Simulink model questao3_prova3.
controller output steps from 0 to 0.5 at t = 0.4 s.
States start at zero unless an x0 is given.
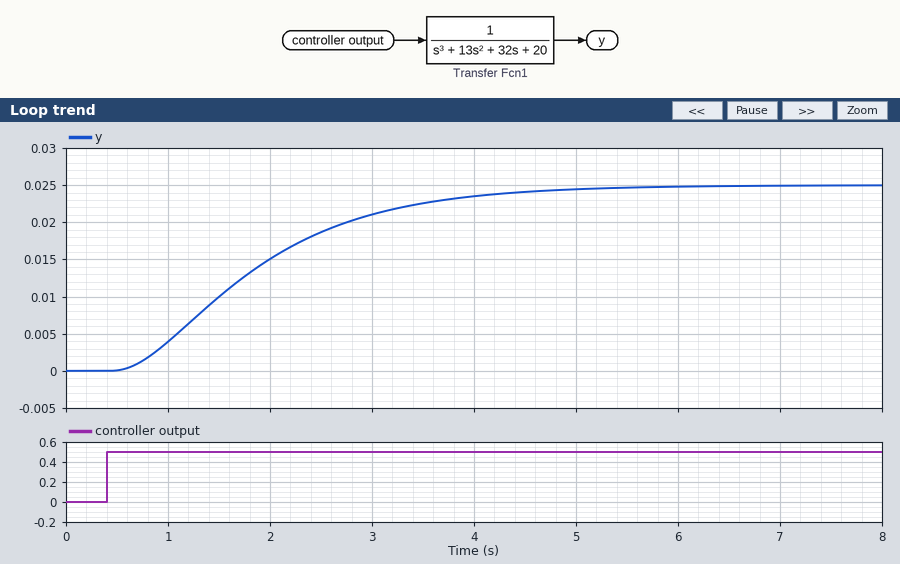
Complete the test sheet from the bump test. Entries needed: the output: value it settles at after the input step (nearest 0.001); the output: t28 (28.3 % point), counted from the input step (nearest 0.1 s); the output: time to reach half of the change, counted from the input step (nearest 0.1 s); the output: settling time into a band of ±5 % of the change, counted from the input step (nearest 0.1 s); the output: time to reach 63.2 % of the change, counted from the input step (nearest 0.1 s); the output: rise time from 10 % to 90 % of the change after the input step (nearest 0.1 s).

0.025
0.9 s
1.3 s
3.8 s
1.7 s
2.6 s
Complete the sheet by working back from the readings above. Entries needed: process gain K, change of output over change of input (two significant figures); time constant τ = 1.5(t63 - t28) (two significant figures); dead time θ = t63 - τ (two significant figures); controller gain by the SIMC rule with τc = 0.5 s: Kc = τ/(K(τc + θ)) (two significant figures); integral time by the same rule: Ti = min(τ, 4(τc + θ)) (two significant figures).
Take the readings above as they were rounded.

0.050
1.2 s
0.50 s
24
1.2 s
